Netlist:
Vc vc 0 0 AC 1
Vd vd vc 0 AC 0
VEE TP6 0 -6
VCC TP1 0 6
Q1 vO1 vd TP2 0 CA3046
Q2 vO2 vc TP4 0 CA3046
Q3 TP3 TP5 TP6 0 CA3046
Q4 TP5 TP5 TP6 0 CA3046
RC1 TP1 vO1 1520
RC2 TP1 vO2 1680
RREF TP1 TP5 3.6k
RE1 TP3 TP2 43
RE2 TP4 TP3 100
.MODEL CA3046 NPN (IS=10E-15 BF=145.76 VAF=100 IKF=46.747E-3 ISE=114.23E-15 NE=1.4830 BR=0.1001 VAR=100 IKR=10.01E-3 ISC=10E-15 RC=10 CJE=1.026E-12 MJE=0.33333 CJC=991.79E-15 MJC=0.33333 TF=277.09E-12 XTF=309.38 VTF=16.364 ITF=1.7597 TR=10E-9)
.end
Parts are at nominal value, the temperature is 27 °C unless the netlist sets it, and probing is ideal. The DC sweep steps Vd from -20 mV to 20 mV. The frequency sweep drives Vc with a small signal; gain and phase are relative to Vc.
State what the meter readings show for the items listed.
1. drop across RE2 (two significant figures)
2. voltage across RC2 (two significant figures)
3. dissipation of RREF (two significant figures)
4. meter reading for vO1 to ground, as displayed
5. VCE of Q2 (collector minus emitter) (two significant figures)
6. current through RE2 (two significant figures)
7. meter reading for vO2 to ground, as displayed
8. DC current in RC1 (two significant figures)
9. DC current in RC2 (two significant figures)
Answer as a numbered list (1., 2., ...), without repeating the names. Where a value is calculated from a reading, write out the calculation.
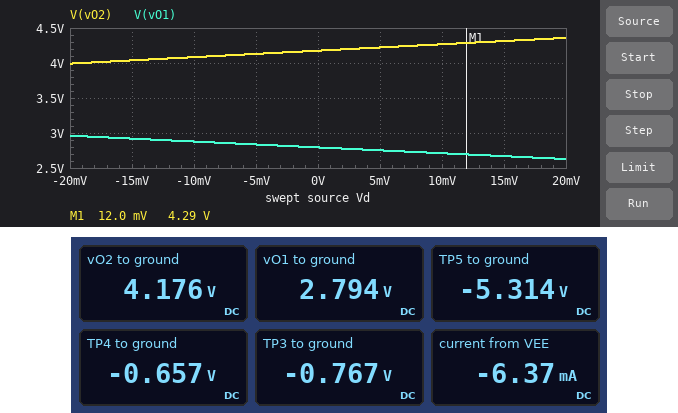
1. -657 mV - (-767 mV) = 110 mV
2. 6 V - 4.176 V = 1.8 V
3. (6 V - (-5.314 V))^2 / 3.6 kΩ = 36 mW
4. 2.794 V
5. 4.176 V - (-657 mV) = 4.8 V
6. (-657 mV - (-767 mV)) / 100 Ω = 1.1 mA
7. 4.176 V
8. (6 V - 2.794 V) / 1.52 kΩ = 2.1 mA
9. (6 V - 4.176 V) / 1.68 kΩ = 1.1 mA
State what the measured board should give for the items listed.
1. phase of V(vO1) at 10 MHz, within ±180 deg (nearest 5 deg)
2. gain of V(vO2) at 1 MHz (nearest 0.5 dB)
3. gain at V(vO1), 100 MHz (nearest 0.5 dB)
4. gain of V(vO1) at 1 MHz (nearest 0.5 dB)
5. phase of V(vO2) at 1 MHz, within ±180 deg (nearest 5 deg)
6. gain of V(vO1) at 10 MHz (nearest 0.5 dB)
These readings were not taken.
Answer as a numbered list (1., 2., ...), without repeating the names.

1. -165 deg
2. -36.0 dB
3. -12.5 dB
4. -30.0 dB
5. 170 deg
6. -29.0 dB
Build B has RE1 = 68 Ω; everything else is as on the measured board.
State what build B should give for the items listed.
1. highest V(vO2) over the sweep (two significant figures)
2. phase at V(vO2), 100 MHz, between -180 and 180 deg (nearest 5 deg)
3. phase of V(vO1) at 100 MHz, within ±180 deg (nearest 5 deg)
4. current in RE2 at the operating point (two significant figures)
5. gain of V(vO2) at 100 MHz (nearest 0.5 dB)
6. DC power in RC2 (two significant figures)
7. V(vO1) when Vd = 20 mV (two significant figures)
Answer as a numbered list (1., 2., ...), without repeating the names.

1. 3.9 V
2. 100 deg
3. 140 deg
4. 1.4 mA
5. -12.5 dB
6. 3.0 mW
7. 3.0 V
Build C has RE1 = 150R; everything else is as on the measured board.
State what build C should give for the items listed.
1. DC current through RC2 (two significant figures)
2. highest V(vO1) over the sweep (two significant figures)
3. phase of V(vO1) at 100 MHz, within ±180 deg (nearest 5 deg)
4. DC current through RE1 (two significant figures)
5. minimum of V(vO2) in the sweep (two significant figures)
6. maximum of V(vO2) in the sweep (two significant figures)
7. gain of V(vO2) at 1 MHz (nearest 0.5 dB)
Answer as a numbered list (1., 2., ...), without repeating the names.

1. 1.9 mA
2. 4.1 V
3. 105 deg
4. 1.3 mA
5. 2.7 V
6. 3.0 V
7. -30.5 dB
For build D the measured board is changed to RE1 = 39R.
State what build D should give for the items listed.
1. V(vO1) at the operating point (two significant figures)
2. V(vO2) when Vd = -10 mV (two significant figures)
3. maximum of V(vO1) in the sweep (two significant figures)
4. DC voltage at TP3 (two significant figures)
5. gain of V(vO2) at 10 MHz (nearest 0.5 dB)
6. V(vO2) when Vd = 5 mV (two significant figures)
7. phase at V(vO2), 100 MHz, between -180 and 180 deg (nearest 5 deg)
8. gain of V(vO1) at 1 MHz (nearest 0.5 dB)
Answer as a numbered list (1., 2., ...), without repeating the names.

1. 2.7 V
2. 4.2 V
3. 2.9 V
4. -760 mV
5. -30.5 dB
6. 4.3 V
7. 85 deg
8. -29.5 dB
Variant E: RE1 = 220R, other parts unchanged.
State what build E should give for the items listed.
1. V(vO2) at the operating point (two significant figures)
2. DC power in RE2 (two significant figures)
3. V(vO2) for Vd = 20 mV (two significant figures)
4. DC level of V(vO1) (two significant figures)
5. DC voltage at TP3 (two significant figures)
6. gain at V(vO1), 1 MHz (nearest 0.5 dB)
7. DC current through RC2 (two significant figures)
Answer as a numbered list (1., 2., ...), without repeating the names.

1. 2.4 V
2. 460 µW
3. 2.5 V
4. 4.4 V
5. -890 mV
6. -36.5 dB
7. 2.1 mA
